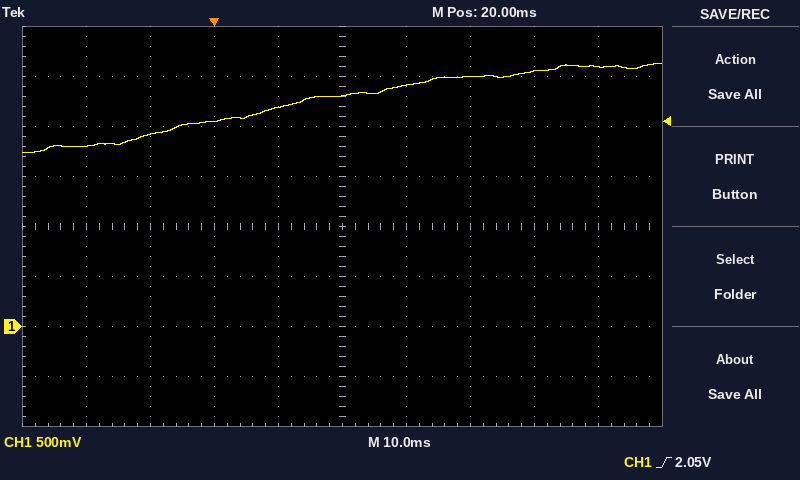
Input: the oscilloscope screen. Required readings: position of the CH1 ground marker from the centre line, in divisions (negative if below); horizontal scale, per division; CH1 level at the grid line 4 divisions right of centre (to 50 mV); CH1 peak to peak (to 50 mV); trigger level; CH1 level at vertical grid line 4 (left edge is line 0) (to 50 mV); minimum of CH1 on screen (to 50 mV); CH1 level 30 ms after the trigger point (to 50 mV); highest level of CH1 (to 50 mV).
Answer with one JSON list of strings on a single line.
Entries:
["-2.0 div", "10 ms", "2.60 V", "900 mV", "2.05 V", "2.20 V", "1.75 V", "2.40 V", "2.65 V"]
